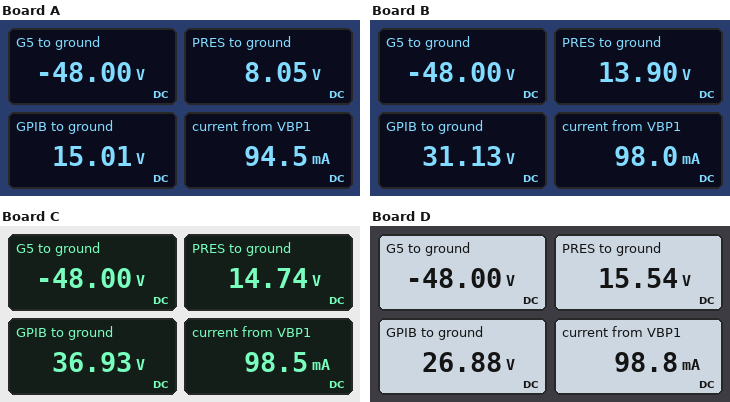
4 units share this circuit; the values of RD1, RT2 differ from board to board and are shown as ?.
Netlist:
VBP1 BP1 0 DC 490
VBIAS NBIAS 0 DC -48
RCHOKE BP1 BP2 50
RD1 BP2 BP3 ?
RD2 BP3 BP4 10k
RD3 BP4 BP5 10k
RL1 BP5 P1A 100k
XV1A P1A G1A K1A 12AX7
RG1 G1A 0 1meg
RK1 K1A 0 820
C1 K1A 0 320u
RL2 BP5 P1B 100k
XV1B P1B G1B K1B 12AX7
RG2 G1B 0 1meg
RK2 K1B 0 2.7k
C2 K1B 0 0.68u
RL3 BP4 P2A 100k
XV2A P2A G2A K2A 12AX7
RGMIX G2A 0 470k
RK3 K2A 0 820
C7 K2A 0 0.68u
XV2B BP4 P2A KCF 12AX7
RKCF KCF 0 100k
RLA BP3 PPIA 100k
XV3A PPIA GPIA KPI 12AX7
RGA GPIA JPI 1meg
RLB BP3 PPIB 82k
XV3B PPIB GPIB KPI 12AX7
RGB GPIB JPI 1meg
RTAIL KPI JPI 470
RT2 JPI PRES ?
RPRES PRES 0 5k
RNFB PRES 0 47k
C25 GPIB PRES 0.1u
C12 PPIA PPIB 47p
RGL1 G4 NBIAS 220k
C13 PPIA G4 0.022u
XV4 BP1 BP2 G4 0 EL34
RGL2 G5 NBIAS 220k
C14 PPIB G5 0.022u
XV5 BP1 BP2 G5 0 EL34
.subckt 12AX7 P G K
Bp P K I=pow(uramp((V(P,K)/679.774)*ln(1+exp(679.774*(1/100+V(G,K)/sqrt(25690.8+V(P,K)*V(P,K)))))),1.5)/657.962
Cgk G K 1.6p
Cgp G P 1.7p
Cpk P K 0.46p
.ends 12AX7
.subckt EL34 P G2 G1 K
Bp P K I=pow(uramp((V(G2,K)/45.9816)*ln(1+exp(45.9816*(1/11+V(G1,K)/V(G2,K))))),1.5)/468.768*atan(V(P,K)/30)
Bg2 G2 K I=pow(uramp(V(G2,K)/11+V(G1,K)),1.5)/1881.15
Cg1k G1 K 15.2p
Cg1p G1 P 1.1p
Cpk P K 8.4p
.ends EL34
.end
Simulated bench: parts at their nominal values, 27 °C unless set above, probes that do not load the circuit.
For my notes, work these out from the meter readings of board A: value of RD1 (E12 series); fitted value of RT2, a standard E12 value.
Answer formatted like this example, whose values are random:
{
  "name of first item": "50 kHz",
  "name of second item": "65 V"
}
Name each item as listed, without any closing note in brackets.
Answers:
{
  "value of RD1": "56 kΩ",
  "fitted value of RT2, a standard E12 value": "3.9 kΩ"
}
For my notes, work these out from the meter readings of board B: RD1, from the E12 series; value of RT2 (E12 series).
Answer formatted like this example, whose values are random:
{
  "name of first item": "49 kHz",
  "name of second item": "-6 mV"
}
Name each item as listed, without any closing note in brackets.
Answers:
{
  "RD1, from the E12 series": "12 kΩ",
  "value of RT2": "5.6 kΩ"
}
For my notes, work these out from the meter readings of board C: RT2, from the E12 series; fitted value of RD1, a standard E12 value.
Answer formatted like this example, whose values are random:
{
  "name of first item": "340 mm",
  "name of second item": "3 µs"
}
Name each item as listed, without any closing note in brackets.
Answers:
{
  "RT2, from the E12 series": "6.8 kΩ",
  "fitted value of RD1, a standard E12 value": "8.2 kΩ"
}
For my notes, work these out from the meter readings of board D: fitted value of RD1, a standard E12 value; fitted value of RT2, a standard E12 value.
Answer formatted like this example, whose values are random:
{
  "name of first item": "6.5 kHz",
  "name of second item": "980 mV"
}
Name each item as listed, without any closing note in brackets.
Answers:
{
  "fitted value of RD1, a standard E12 value": "6.8 kΩ",
  "fitted value of RT2, a standard E12 value": "3.3 kΩ"
}
